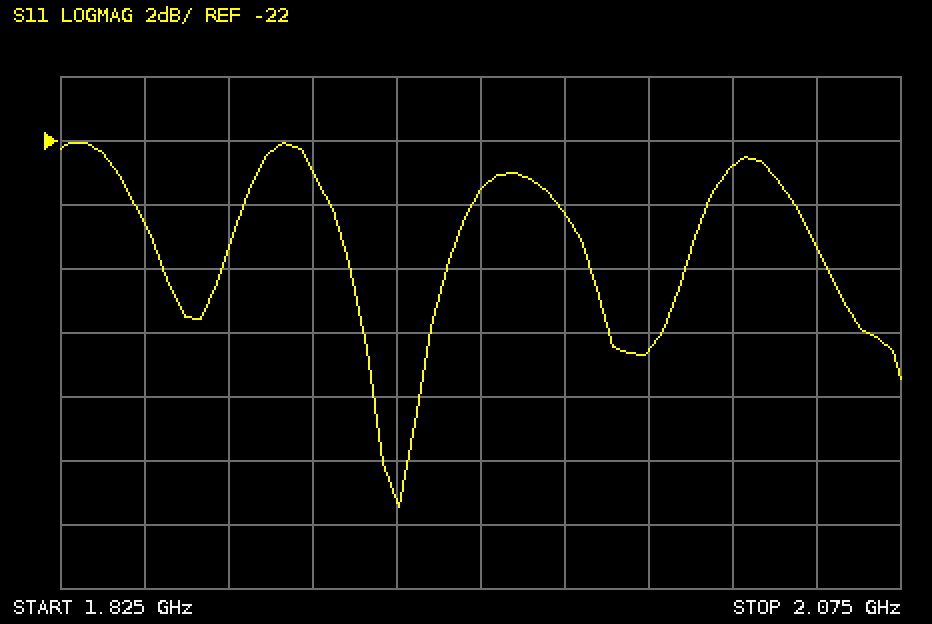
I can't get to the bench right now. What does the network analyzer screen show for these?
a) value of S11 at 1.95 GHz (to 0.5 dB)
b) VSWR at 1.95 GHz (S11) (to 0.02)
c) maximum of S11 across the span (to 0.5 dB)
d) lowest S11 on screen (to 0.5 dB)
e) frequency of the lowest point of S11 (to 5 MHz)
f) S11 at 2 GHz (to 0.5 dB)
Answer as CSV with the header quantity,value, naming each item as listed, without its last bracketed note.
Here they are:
quantity,value
value of S11 at 1.95 GHz,-23.5 dB
VSWR at 1.95 GHz (S11),1.14
maximum of S11 across the span,-22.0 dB
lowest S11 on screen,-33.5 dB
frequency of the lowest point of S11,1.925 GHz
S11 at 2 GHz,-28.5 dB
